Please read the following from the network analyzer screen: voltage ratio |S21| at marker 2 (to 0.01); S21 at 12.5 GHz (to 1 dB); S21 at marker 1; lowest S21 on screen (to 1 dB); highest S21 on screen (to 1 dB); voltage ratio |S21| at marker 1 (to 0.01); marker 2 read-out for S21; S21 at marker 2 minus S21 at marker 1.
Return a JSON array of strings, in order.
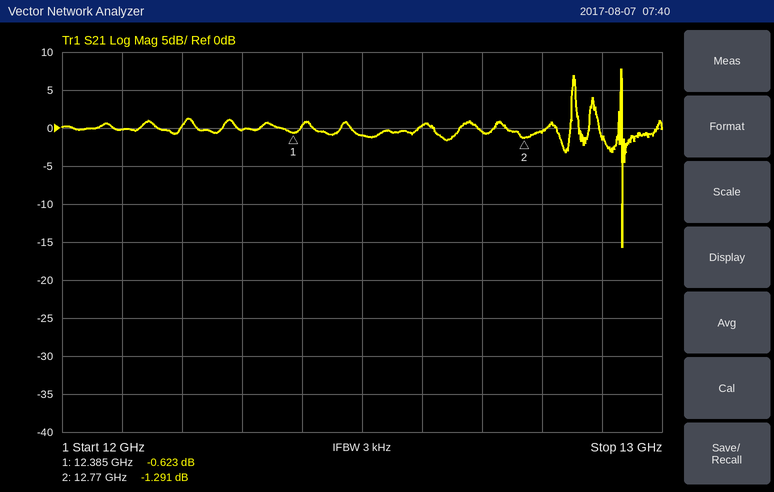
["0.86", "-1 dB", "-0.623 dB", "-16 dB", "8 dB", "0.93", "-1.291 dB", "-0.668 dB"]
